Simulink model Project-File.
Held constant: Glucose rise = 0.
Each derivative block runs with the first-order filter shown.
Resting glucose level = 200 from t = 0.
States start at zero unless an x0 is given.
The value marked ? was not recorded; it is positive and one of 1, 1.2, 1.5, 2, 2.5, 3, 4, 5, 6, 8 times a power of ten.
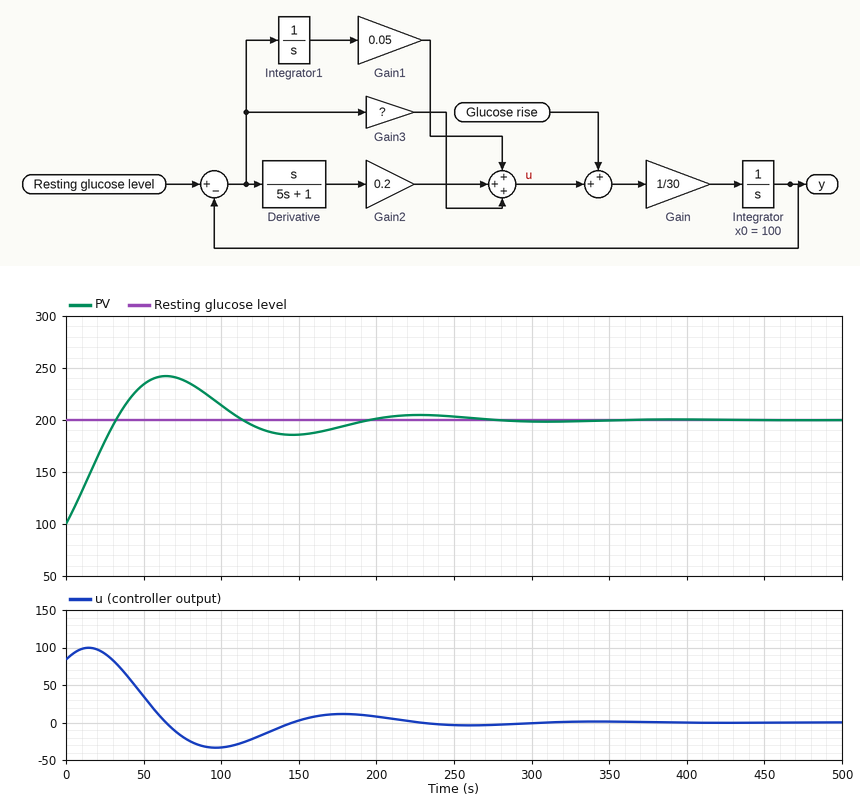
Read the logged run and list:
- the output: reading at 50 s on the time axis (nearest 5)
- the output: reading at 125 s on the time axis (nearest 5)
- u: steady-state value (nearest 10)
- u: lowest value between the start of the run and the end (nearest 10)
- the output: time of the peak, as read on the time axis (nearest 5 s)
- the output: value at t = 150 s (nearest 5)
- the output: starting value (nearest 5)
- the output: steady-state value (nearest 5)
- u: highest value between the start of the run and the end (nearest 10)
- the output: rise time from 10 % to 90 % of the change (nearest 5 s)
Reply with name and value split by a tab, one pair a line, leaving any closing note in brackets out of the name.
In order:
the output: reading at 50 s on the time axis	235
the output: reading at 125 s on the time axis	190
u: steady-state value	0
u: lowest value between the start of the run and the end	-30
the output: time of the peak, as read on the time axis	65 s
the output: value at t = 150 s	185
the output: starting value	100
the output: steady-state value	200
u: highest value between the start of the run and the end	100
the output: rise time from 10 % to 90 % of the change	25 s
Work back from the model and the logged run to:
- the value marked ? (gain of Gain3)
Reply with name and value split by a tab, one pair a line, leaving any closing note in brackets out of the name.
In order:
the value marked ?	0.8
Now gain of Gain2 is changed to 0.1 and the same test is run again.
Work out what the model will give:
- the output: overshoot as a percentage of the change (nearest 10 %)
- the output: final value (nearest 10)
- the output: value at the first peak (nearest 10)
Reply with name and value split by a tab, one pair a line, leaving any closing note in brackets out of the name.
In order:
the output: overshoot as a percentage of the change	40 %
the output: final value	200
the output: value at the first peak	240
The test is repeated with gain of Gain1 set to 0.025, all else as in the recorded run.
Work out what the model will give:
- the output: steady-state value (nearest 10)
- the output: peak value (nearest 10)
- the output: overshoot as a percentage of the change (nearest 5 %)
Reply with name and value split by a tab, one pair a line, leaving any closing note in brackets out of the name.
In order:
the output: steady-state value	200
the output: peak value	230
the output: overshoot as a percentage of the change	30 %
